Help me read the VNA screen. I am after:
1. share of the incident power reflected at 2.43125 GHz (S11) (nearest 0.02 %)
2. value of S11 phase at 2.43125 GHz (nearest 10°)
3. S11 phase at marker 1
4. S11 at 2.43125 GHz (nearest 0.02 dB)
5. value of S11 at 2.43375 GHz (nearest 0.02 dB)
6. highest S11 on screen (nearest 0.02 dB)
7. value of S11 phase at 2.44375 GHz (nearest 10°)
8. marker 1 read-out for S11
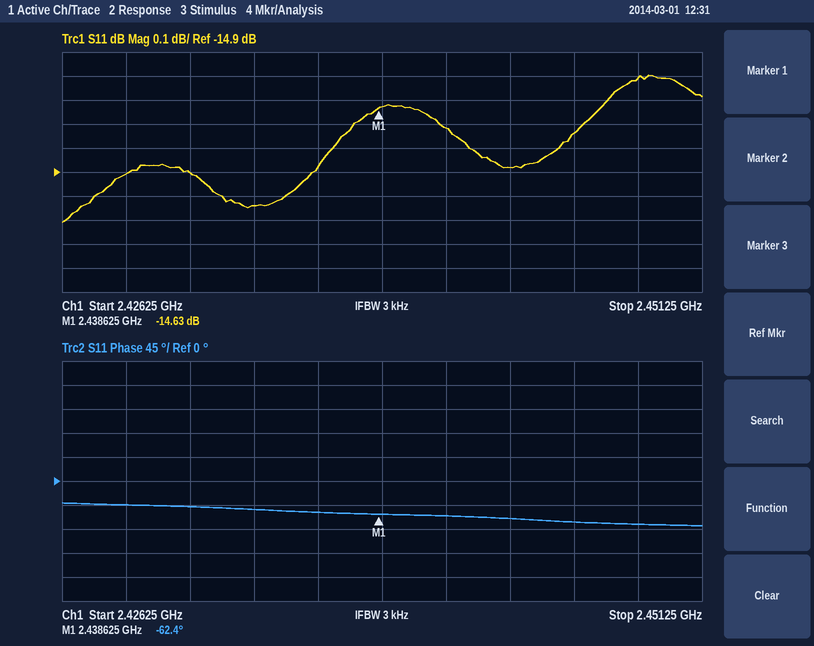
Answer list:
3.24 %
-50°
-62.4°
-14.90 dB
-15.04 dB
-14.50 dB
-70°
-14.63 dB
